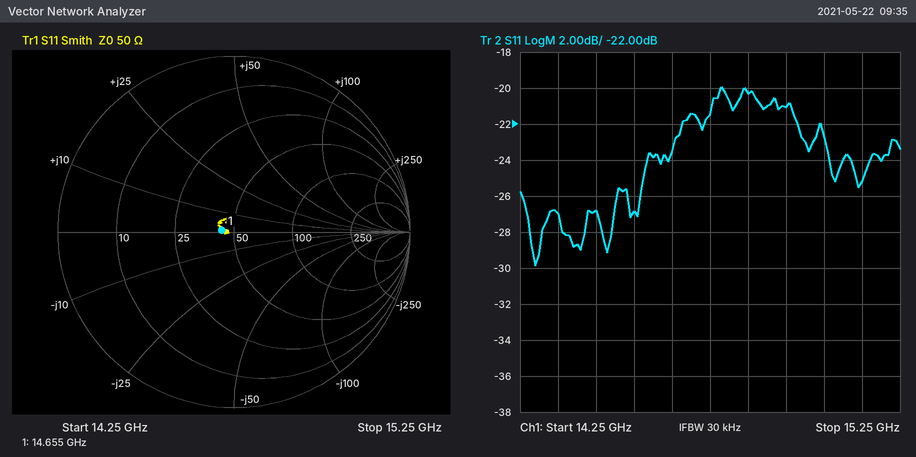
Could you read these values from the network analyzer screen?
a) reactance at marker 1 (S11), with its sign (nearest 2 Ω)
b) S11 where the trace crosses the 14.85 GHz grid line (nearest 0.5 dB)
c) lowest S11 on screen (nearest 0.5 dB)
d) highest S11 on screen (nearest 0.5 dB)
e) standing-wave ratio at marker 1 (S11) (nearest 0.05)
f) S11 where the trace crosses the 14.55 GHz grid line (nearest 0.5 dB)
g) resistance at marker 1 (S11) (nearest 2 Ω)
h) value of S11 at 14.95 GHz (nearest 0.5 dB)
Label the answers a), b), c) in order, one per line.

a) 0 Ω
b) -20.5 dB
c) -30.0 dB
d) -20.0 dB
e) 1.15
f) -27.0 dB
g) 44 Ω
h) -21.0 dB
